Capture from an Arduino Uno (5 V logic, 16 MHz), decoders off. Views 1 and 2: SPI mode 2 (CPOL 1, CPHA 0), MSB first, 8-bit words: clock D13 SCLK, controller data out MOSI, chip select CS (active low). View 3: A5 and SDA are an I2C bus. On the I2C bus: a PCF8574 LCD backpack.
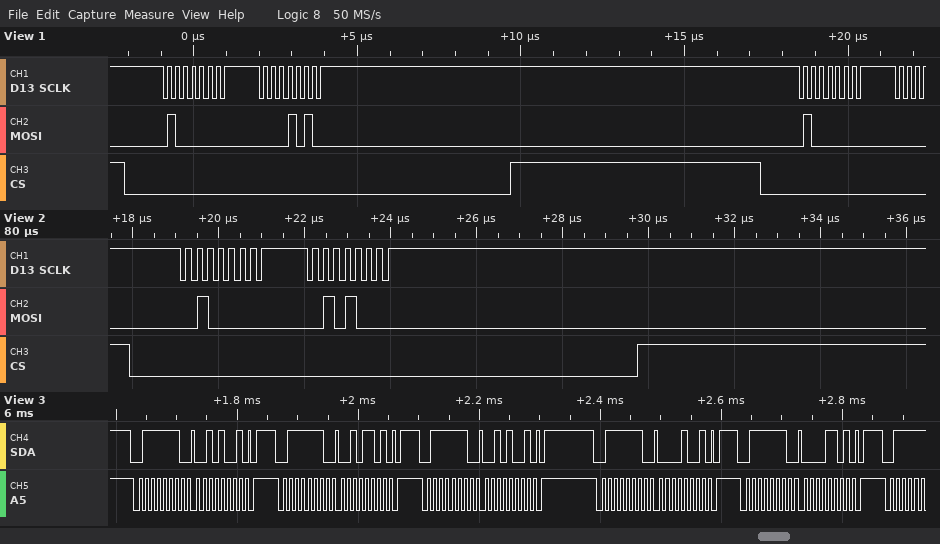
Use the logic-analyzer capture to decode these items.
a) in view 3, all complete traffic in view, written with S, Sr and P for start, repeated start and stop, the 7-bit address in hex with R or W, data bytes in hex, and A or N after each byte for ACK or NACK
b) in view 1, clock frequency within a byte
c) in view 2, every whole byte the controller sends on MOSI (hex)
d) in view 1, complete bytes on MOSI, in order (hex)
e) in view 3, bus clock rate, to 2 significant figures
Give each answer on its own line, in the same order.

S 3FW A 29 A P S 3FW A 2D A P S 3FW A 29 A P S 3FW A 09 A P S 3FW A 0D A P
4 MHz
20 28
40 0A 40
100 kHz
